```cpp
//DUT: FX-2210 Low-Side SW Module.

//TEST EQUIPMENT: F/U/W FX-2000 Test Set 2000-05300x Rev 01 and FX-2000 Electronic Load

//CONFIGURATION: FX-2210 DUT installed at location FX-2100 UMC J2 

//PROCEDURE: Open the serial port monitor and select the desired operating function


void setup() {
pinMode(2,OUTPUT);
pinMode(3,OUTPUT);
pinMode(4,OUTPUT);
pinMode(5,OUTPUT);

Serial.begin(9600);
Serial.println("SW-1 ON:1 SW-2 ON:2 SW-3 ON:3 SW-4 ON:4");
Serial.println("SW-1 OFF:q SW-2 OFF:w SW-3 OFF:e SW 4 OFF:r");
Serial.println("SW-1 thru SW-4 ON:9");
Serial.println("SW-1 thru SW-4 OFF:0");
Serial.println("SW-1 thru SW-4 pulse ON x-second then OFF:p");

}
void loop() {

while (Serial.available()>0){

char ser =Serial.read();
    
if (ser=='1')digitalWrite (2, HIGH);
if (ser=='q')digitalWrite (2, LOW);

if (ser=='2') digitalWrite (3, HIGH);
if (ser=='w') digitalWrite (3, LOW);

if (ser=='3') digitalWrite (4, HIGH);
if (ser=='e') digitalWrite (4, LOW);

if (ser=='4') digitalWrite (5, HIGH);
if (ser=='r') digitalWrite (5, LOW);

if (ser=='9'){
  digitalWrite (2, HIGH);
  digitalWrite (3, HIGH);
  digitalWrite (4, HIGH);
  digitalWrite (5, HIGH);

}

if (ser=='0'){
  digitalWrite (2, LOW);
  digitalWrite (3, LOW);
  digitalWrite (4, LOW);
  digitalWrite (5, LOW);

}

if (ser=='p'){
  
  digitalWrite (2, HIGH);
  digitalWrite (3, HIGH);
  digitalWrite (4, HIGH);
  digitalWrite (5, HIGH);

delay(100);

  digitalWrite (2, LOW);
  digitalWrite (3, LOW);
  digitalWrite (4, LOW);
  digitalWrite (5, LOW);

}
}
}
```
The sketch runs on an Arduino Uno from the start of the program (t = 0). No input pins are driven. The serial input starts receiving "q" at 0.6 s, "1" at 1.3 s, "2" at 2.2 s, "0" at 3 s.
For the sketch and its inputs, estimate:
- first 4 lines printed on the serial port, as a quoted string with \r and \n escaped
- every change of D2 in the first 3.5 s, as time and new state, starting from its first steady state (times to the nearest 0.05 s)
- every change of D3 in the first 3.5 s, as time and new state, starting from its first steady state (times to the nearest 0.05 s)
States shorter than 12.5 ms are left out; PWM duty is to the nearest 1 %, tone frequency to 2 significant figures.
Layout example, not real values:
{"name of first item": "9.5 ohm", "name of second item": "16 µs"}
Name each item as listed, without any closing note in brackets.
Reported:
{"first 4 lines printed on the serial port, as a quoted string with \\r and \\n escaped": "\"SW-1 ON:1 SW-2 ON:2 SW-3 ON:3 SW-4 ON:4\\r\\nSW-1 OFF:q SW-2 OFF:w SW-3 OFF:e SW 4 OFF:r\\r\\nSW-1 thru SW-4 ON:9\\r\\nSW-1 thru SW-4 OFF:0\\r\\n\"", "every change of D2 in the first 3.5 s, as time and new state, starting from its first steady state": "0 s low; 1.3 s high; 3 s low", "every change of D3 in the first 3.5 s, as time and new state, starting from its first steady state": "0 s low; 2.2 s high; 3 s low"}
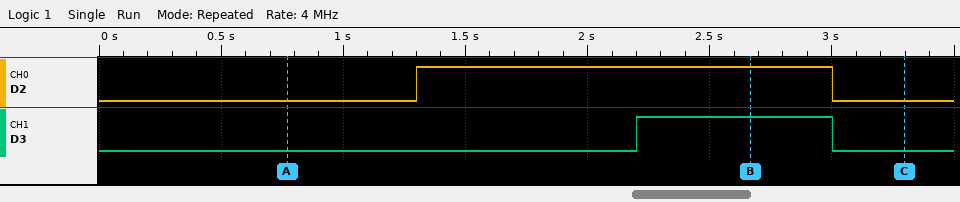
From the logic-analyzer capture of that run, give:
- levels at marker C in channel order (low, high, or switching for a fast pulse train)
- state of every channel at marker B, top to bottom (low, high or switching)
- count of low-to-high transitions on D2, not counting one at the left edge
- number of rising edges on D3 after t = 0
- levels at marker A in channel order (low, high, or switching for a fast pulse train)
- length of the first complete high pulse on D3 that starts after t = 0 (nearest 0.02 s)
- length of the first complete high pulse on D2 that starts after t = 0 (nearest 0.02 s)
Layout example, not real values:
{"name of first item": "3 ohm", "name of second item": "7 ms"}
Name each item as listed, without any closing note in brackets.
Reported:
{"levels at marker C in channel order": "D2 low, D3 low", "state of every channel at marker B, top to bottom": "D2 high, D3 high", "count of low-to-high transitions on D2, not counting one at the left edge": "1", "number of rising edges on D3 after t = 0": "1", "levels at marker A in channel order": "D2 low, D3 low", "length of the first complete high pulse on D3 that starts after t = 0": "0.80 s", "length of the first complete high pulse on D2 that starts after t = 0": "1.70 s"}
